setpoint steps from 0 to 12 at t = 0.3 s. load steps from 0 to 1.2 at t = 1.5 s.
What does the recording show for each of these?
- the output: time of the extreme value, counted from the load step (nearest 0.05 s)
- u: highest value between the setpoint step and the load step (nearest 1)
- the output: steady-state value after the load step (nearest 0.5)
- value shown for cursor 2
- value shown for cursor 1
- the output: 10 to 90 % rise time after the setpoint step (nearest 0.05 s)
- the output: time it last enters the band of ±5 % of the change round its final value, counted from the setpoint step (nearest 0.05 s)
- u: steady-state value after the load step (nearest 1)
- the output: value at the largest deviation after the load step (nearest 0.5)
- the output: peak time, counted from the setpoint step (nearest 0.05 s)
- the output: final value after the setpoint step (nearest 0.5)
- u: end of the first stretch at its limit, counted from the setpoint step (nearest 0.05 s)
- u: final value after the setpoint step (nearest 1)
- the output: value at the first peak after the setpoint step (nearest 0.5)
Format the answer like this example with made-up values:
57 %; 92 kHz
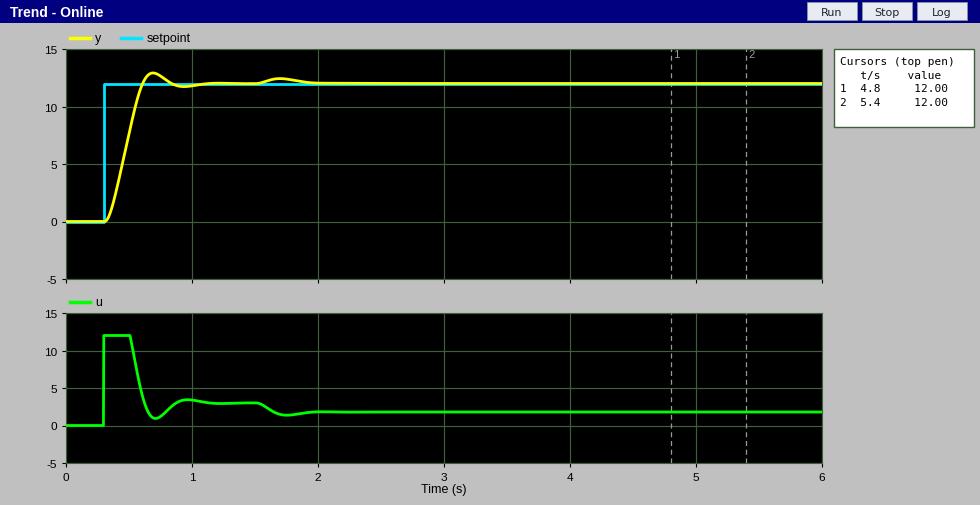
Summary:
0.20 s; 12; 12.0; 12.00; 12.00; 0.20 s; 0.45 s; 2; 12.5; 0.40 s; 12.0; 0.20 s; 3; 13.0
